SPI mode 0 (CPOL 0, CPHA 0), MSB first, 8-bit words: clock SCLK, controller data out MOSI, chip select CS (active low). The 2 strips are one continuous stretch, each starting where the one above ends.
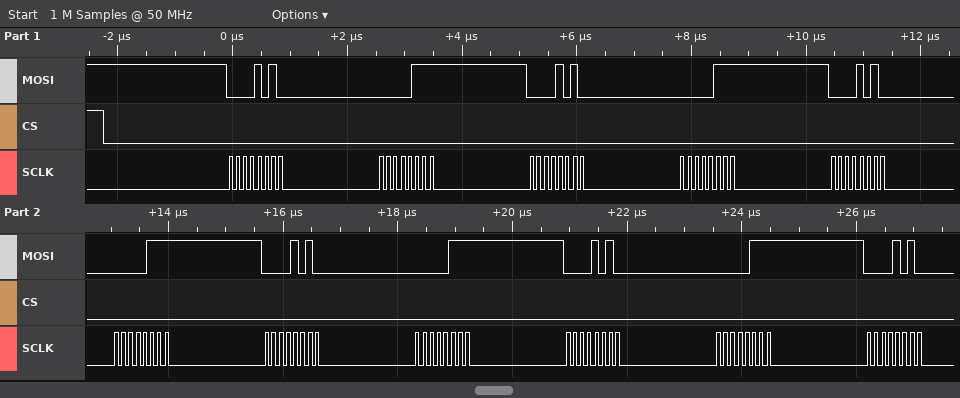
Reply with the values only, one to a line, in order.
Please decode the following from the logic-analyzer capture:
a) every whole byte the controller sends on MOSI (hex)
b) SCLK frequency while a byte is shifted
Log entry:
0A 07 0A 07 0A 07 0A 07 0A 07 0A
8 MHz
